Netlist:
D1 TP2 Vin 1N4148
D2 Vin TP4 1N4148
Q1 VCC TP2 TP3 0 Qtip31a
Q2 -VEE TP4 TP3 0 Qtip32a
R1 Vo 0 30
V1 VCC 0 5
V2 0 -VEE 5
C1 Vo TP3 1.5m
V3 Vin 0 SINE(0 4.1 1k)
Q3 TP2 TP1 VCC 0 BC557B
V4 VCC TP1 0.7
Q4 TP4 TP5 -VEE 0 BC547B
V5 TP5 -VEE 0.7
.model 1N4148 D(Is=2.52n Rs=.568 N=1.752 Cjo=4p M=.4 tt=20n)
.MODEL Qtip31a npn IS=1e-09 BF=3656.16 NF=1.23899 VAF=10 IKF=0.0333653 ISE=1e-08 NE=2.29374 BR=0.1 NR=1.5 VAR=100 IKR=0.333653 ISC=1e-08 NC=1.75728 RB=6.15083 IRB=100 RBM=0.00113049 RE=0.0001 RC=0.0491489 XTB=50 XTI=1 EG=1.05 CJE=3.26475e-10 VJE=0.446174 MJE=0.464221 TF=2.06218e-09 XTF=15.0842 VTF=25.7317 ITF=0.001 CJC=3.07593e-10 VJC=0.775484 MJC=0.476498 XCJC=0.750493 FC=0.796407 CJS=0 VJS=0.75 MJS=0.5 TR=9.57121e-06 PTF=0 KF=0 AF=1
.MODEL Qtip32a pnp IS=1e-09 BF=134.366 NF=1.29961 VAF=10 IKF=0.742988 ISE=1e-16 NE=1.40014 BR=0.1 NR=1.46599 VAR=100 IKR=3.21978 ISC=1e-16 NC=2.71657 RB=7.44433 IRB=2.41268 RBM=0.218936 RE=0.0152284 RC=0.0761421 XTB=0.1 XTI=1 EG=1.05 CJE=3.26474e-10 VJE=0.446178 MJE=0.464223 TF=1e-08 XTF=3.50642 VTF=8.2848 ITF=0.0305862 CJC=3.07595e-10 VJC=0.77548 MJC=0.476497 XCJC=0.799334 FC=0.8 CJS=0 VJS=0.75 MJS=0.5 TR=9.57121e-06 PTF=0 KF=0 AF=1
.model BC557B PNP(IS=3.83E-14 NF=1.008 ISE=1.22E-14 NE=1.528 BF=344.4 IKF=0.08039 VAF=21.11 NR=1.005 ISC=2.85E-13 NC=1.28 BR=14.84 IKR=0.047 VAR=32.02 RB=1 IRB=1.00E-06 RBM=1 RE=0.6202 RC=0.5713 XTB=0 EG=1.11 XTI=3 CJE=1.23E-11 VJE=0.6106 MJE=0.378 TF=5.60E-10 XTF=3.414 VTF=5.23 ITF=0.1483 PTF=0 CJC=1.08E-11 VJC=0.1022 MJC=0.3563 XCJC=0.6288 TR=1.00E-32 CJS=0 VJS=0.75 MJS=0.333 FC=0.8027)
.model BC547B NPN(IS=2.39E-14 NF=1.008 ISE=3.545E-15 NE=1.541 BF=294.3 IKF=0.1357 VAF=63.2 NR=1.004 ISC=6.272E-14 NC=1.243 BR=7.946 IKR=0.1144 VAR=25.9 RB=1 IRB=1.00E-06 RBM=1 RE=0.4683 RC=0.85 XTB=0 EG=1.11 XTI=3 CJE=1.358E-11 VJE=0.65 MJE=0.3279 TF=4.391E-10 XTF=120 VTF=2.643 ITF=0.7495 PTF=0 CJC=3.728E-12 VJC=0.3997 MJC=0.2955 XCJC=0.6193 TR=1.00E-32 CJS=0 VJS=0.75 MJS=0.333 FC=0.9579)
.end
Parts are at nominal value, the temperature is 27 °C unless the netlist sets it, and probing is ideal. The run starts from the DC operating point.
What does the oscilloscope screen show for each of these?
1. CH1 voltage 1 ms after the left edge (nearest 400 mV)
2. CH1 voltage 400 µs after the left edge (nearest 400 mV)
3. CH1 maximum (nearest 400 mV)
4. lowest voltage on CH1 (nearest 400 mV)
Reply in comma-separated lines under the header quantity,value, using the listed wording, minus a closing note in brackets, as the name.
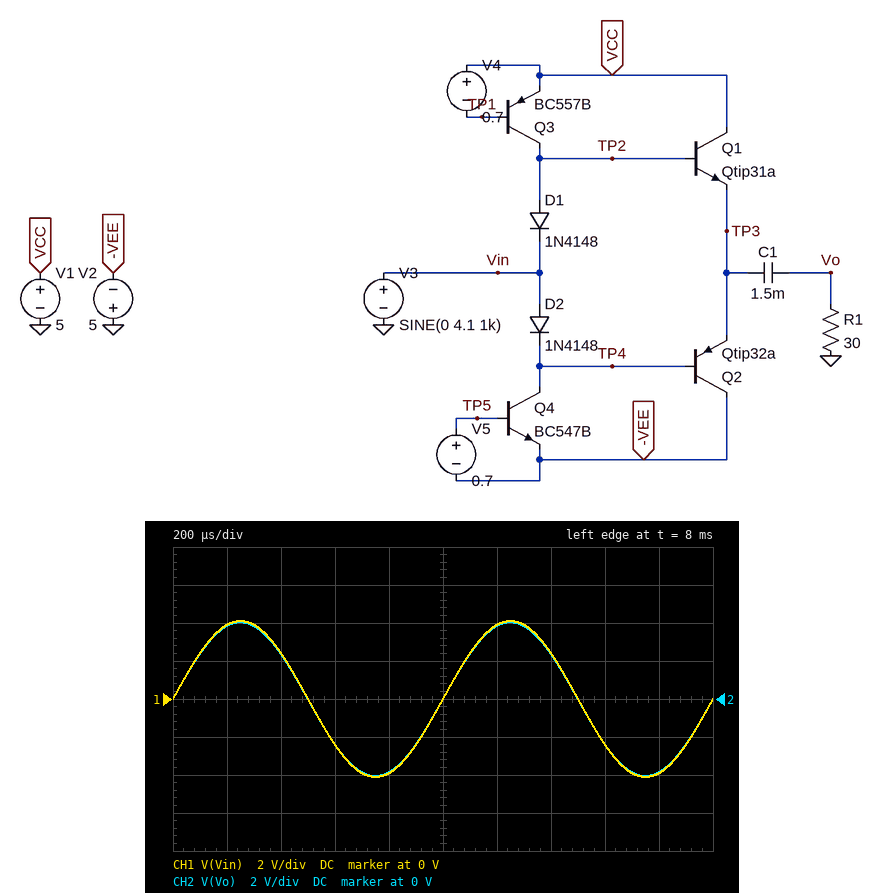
quantity,value
CH1 voltage 1 ms after the left edge,0 V
CH1 voltage 400 µs after the left edge,2.4 V
CH1 maximum,4.0 V
lowest voltage on CH1,-4.0 V
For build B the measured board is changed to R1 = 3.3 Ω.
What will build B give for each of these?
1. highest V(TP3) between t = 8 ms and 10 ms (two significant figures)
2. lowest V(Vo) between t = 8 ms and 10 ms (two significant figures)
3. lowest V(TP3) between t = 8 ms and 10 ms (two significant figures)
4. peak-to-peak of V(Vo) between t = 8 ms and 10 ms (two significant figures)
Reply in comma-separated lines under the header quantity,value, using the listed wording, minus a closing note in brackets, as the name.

quantity,value
highest V(TP3) between t = 8 ms and 10 ms,3.5 V
lowest V(Vo) between t = 8 ms and 10 ms,-2.5 V
lowest V(TP3) between t = 8 ms and 10 ms,-2.3 V
peak-to-peak of V(Vo) between t = 8 ms and 10 ms,5.8 V
